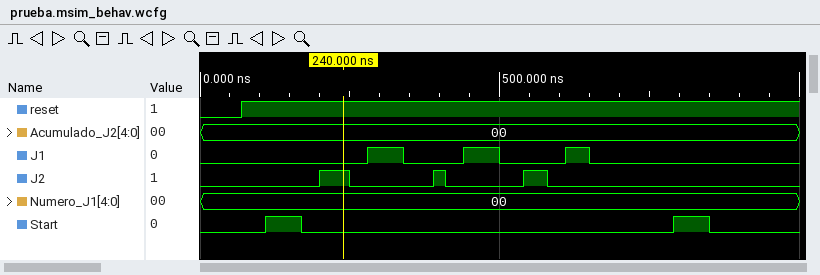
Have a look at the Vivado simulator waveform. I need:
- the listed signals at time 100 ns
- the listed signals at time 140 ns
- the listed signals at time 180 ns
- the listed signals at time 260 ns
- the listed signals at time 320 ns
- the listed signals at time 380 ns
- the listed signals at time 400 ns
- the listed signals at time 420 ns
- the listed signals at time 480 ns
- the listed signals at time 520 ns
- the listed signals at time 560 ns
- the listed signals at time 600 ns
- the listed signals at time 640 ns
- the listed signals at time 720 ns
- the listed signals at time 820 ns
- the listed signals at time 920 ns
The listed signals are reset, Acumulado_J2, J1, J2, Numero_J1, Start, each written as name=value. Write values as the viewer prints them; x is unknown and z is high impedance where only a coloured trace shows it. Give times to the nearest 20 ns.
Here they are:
reset=1, Acumulado_J2=00, J1=0, J2=0, Numero_J1=00, Start=0
reset=1, Acumulado_J2=00, J1=0, J2=0, Numero_J1=00, Start=1
reset=1, Acumulado_J2=00, J1=0, J2=0, Numero_J1=00, Start=0
reset=1, Acumulado_J2=00, J1=0, J2=0, Numero_J1=00, Start=0
reset=1, Acumulado_J2=00, J1=1, J2=0, Numero_J1=00, Start=0
reset=1, Acumulado_J2=00, J1=0, J2=0, Numero_J1=00, Start=0
reset=1, Acumulado_J2=00, J1=0, J2=1, Numero_J1=00, Start=0
reset=1, Acumulado_J2=00, J1=0, J2=0, Numero_J1=00, Start=0
reset=1, Acumulado_J2=00, J1=1, J2=0, Numero_J1=00, Start=0
reset=1, Acumulado_J2=00, J1=0, J2=0, Numero_J1=00, Start=0
reset=1, Acumulado_J2=00, J1=0, J2=1, Numero_J1=00, Start=0
reset=1, Acumulado_J2=00, J1=0, J2=0, Numero_J1=00, Start=0
reset=1, Acumulado_J2=00, J1=1, J2=0, Numero_J1=00, Start=0
reset=1, Acumulado_J2=00, J1=0, J2=0, Numero_J1=00, Start=0
reset=1, Acumulado_J2=00, J1=0, J2=0, Numero_J1=00, Start=1
reset=1, Acumulado_J2=00, J1=0, J2=0, Numero_J1=00, Start=0
